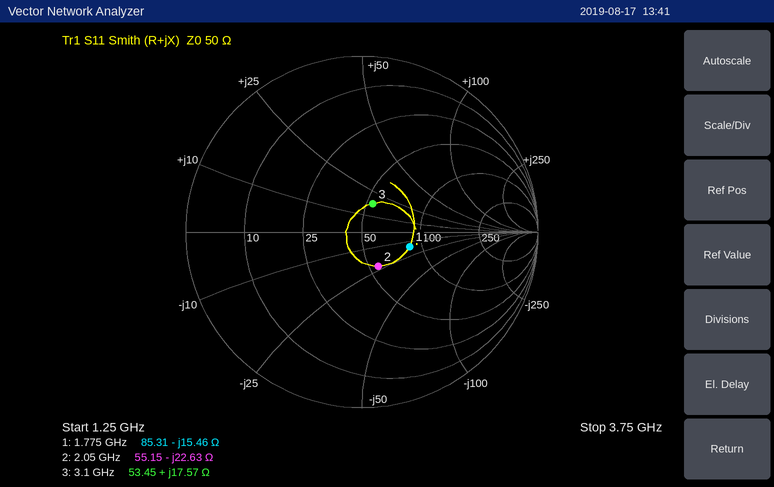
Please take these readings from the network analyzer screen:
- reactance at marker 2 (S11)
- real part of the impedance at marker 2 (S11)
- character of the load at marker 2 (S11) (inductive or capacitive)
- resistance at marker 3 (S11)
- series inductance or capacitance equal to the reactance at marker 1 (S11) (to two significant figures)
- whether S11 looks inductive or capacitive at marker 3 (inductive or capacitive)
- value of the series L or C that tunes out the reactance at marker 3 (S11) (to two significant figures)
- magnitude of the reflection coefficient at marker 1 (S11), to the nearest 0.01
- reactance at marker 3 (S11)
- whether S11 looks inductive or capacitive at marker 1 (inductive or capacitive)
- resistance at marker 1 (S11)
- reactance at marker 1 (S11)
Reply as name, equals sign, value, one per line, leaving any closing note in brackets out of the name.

reactance at marker 2 = -22.63 Ω
real part of the impedance at marker 2 = 55.15 Ω
character of the load at marker 2 (S11) = capacitive
resistance at marker 3 = 53.45 Ω
series inductance or capacitance equal to the reactance at marker 1 (S11) = 5.8 pF
whether S11 looks inductive or capacitive at marker 3 = inductive
value of the series L or C that tunes out the reactance at marker 3 (S11) = 2.9 pF
magnitude of the reflection coefficient at marker 1 (S11), to the nearest 0.01 = 0.28
reactance at marker 3 = +17.57 Ω
whether S11 looks inductive or capacitive at marker 1 = capacitive
resistance at marker 1 = 85.31 Ω
reactance at marker 1 = -15.46 Ω
